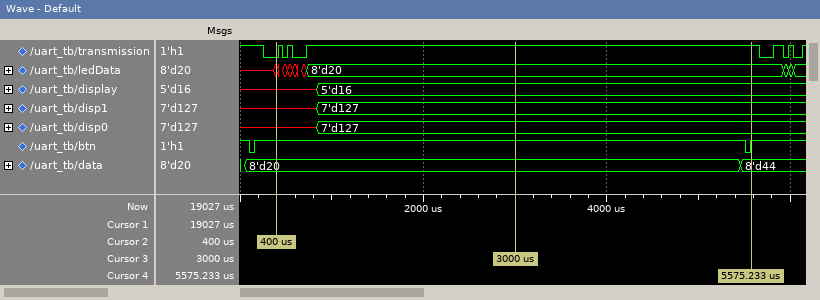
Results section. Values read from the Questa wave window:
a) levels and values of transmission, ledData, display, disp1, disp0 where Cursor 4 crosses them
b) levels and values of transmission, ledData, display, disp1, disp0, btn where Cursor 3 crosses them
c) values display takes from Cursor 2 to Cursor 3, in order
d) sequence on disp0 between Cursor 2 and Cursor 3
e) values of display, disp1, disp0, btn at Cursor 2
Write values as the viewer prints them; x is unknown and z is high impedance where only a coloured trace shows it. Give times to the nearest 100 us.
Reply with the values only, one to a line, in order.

transmission=1, ledData=8'd20, display=5'd16, disp1=7'd127, disp0=7'd127
transmission=1, ledData=8'd20, display=5'd16, disp1=7'd127, disp0=7'd127, btn=1
x, 5'd16
x, 7'd127
display=x, disp1=x, disp0=x, btn=1
